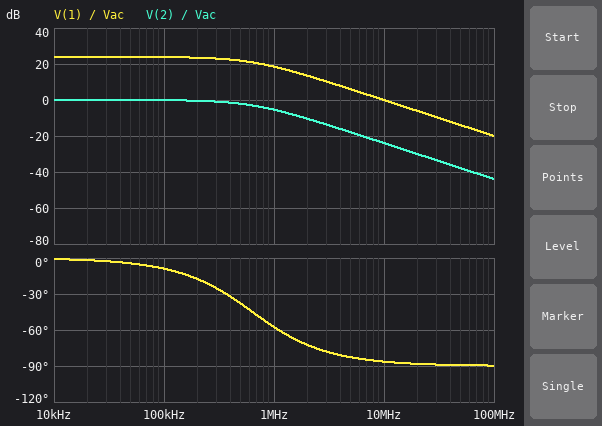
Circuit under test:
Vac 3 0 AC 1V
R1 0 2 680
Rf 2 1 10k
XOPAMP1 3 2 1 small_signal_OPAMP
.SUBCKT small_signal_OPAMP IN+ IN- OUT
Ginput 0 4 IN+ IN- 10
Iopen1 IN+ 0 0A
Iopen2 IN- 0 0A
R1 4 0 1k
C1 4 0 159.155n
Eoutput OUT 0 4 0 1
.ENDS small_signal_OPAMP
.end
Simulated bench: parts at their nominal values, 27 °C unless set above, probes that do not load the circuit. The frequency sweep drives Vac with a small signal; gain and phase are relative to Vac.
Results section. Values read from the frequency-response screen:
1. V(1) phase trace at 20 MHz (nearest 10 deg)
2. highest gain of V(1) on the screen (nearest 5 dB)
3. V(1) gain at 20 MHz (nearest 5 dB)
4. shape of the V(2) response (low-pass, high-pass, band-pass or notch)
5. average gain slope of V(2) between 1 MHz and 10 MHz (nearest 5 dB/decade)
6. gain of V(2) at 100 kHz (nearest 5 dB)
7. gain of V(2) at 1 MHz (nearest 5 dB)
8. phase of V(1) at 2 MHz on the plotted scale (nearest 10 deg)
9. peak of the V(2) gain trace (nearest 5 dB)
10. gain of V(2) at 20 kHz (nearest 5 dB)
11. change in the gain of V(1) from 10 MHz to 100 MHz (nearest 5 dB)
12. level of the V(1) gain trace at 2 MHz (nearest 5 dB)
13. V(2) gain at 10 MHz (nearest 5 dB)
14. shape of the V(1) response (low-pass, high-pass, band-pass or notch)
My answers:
-90 deg
25 dB
-5 dB
low-pass
-20 dB/decade
0 dB
-5 dB
-70 deg
0 dB
0 dB
-20 dB
15 dB
-25 dB
low-pass
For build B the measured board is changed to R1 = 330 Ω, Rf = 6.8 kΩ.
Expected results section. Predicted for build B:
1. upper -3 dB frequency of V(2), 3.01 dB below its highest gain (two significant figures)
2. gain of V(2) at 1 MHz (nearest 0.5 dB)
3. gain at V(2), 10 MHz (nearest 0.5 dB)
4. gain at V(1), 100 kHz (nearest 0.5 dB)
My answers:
460 kHz
-7.5 dB
-26.5 dB
26.5 dB
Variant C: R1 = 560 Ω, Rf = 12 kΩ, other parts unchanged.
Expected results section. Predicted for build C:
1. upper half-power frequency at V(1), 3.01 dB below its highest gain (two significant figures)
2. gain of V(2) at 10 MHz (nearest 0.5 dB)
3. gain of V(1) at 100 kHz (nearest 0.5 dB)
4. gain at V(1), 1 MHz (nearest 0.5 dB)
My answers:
450 kHz
-27.0 dB
27.0 dB
19.0 dB
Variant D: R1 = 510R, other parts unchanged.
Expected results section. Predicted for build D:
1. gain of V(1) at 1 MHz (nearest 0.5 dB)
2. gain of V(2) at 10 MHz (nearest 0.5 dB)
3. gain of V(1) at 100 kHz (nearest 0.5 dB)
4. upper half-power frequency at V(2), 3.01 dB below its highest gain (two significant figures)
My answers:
19.0 dB
-26.5 dB
26.0 dB
490 kHz
